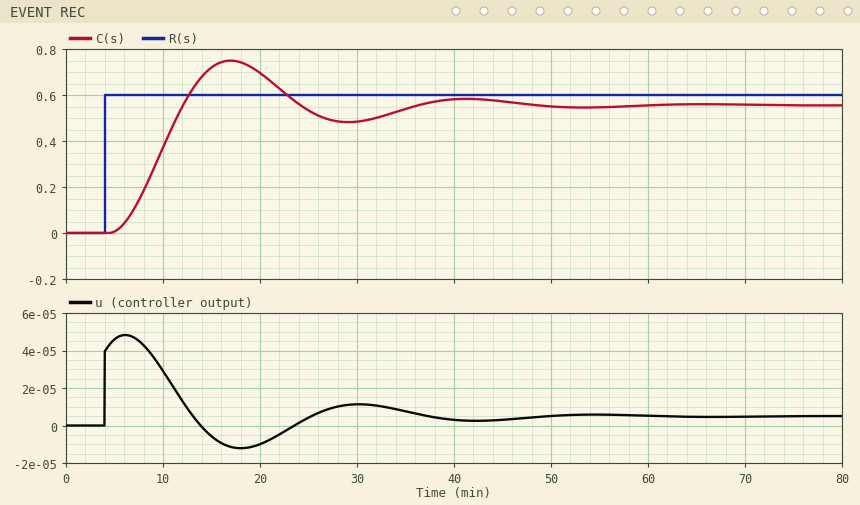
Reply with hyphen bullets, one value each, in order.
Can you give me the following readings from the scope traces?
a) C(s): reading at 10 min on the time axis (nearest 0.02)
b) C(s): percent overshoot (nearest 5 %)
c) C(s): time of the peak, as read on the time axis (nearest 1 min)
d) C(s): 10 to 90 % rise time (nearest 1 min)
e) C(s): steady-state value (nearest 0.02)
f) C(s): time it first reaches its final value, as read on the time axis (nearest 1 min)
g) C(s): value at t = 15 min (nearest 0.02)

- 0.38
- 35 %
- 17 min
- 5 min
- 0.56
- 12 min
- 0.72
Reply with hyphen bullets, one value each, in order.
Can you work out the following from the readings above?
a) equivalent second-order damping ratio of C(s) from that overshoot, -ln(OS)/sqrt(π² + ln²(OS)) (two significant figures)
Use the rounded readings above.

- 0.32
